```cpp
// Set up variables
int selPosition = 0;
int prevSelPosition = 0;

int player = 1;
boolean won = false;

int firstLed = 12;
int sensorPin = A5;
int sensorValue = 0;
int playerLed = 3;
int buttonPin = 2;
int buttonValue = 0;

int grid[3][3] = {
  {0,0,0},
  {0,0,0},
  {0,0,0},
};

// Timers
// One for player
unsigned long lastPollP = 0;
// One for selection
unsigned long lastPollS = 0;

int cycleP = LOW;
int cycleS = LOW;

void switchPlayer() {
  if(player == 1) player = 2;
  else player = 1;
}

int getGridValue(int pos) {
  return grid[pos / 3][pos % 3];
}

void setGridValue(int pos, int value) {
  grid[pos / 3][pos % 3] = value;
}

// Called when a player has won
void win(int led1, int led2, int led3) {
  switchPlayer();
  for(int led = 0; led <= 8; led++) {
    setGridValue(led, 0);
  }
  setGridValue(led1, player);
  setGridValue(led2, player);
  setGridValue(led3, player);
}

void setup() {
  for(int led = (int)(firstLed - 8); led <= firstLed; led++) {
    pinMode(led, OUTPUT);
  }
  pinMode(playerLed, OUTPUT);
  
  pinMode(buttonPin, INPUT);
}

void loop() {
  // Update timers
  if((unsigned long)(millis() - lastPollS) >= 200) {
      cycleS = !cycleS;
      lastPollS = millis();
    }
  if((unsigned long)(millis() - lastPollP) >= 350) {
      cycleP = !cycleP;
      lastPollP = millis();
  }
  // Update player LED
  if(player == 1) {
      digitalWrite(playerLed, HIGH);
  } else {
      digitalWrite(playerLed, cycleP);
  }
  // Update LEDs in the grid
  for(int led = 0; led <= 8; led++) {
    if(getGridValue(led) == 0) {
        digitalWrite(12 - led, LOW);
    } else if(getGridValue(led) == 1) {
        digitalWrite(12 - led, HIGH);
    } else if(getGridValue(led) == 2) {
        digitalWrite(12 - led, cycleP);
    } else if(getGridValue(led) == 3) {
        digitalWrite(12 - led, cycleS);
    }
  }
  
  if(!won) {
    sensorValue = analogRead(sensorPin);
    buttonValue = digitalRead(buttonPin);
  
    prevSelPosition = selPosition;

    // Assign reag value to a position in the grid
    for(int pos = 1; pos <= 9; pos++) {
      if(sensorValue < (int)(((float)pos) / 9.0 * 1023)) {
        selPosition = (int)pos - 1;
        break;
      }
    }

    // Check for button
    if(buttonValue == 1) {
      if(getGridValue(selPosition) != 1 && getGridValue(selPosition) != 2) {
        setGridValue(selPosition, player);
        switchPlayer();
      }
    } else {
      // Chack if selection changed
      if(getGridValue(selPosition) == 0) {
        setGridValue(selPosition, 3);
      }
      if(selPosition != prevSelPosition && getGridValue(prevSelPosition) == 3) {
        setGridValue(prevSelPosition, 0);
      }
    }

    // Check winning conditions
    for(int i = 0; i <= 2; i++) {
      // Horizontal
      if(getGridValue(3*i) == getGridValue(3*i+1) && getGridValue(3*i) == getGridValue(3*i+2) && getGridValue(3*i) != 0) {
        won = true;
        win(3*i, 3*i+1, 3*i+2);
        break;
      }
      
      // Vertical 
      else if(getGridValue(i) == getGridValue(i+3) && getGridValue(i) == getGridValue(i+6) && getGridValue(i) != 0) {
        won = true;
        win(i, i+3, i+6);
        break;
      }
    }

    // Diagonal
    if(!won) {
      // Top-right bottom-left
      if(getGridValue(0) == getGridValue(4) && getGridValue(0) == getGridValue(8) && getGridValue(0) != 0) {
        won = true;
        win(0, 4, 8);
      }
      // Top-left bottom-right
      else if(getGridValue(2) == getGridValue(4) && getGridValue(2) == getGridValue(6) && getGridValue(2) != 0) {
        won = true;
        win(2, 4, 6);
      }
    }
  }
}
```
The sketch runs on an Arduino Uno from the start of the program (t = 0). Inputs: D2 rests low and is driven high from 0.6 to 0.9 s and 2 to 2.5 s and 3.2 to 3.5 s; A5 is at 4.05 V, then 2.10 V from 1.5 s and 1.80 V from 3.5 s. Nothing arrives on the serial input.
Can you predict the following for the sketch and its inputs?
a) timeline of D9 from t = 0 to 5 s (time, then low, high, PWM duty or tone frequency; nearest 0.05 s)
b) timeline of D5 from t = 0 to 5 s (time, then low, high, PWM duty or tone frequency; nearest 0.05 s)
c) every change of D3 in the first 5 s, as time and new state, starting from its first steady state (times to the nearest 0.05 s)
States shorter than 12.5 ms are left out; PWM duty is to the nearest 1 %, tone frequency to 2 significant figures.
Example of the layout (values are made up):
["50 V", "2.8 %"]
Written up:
["0 s low; 1.5 s high; 1.6 s low; 1.8 s high; 2.1 s low; 2.45 s high; 2.8 s low; 3.15 s high; 3.5 s low; 3.85 s high; 4.2 s low; 4.55 s high; 4.9 s low", "0 s low; 0.2 s high; 0.4 s low; 0.6 s high", "0 s high; 0.7 s low; 1.05 s high; 1.4 s low; 1.75 s high"]
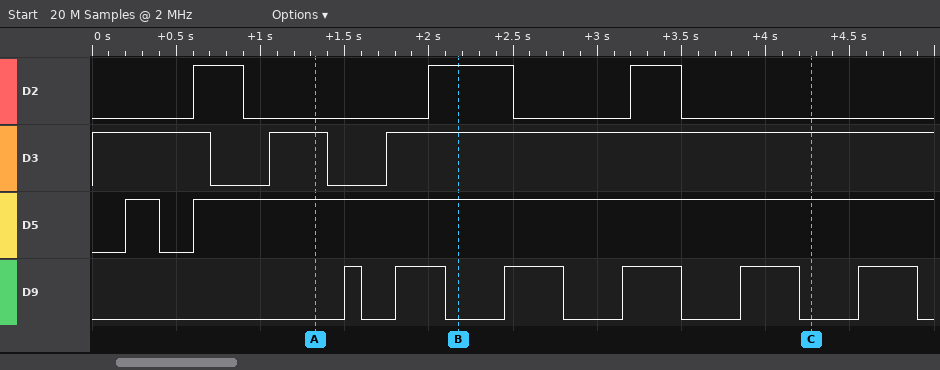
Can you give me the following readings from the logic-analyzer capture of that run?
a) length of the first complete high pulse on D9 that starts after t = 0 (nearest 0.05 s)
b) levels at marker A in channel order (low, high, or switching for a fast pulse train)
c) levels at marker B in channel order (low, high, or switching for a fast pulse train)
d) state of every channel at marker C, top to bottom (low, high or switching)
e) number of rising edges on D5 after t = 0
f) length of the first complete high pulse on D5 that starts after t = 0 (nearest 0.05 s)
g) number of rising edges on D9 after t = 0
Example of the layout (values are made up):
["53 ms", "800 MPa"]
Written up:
["0.10 s", "D2 low, D3 high, D5 high, D9 low", "D2 high, D3 high, D5 high, D9 low", "D2 low, D3 high, D5 high, D9 low", "2", "0.20 s", "6"]
